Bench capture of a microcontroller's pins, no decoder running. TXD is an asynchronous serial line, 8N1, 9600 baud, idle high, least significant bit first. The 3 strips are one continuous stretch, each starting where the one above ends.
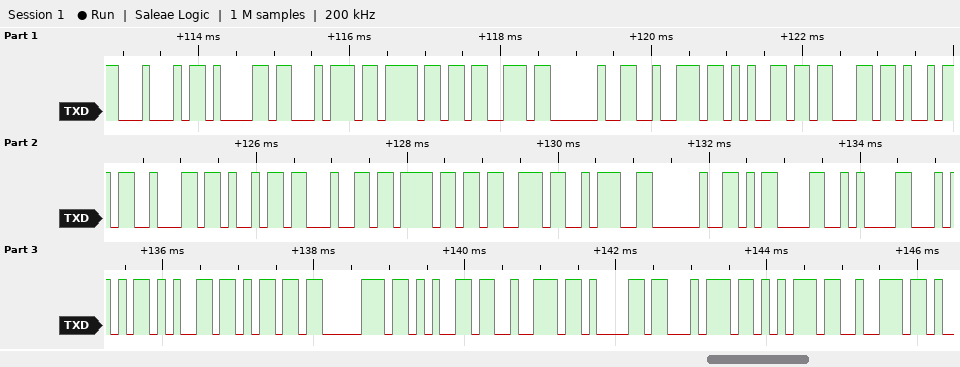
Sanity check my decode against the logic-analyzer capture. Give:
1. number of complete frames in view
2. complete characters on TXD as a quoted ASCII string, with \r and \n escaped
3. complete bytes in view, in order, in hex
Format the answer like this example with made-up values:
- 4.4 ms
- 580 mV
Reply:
- 29
- "Datos recibidos: \r\nTemperatur"
- 44 61 74 6F 73 20 72 65 63 69 62 69 64 6F 73 3A 20 0D 0A 54 65 6D 70 65 72 61 74 75 72
